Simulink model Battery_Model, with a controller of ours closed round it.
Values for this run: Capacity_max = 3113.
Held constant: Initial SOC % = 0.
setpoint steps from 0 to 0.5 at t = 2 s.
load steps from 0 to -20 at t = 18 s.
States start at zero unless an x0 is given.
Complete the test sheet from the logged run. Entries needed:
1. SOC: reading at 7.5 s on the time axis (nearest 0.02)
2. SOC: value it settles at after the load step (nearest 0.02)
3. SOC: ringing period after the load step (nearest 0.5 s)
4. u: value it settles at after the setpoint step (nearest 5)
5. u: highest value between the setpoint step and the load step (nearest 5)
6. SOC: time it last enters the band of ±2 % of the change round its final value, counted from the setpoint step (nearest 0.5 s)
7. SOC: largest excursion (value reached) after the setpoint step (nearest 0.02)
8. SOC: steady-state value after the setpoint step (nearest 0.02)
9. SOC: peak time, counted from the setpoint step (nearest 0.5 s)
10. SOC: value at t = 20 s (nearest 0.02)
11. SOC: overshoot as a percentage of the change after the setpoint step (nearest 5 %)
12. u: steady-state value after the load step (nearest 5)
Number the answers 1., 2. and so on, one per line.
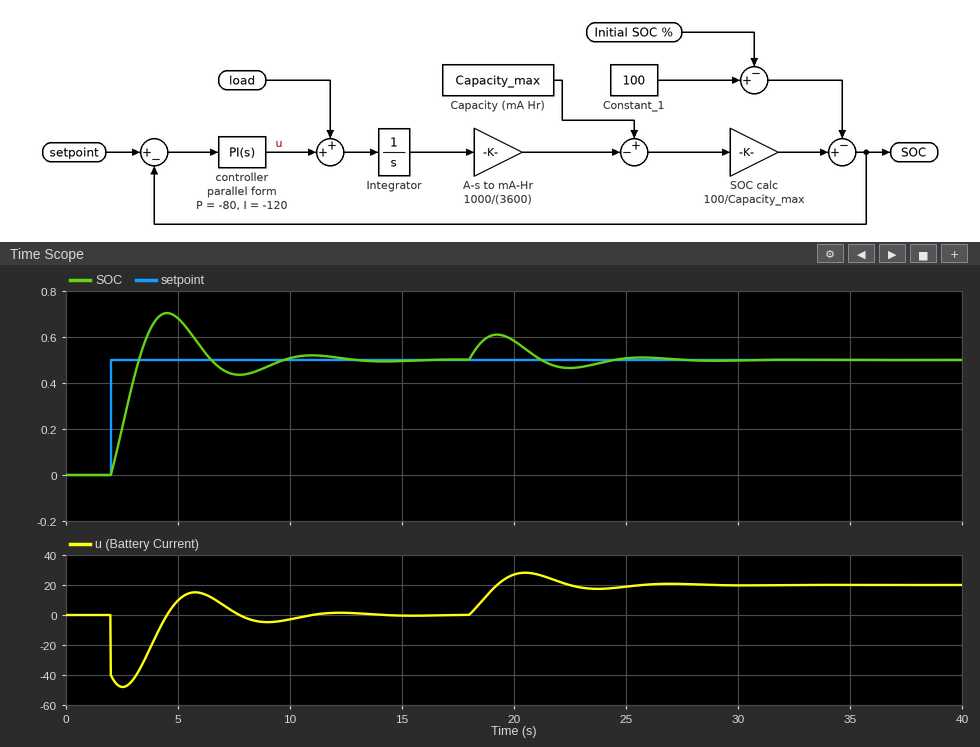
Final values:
1. 0.44
2. 0.50
3. 6.5 s
4. 0
5. 15
6. 10.0 s
7. 0.70
8. 0.50
9. 2.5 s
10. 0.58
11. 40 %
12. 20
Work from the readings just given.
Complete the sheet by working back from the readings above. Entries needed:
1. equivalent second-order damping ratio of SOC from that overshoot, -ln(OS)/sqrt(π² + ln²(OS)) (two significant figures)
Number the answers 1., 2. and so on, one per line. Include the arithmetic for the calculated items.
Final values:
1. ln(0.4) = -0.916; 0.916 / sqrt(9.870 + 0.840) = 0.28
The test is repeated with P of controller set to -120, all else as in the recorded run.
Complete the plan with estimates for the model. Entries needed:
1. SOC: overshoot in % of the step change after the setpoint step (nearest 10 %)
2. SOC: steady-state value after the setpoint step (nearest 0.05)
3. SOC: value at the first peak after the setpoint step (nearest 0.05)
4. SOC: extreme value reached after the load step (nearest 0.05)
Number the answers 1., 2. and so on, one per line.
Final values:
1. 30 %
2. 0.50
3. 0.65
4. 0.60
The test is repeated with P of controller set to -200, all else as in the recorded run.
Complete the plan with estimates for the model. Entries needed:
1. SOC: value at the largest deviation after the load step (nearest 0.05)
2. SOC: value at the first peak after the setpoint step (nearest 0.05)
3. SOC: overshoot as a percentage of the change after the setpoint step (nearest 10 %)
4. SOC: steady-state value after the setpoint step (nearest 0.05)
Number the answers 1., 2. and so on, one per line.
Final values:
1. 0.55
2. 0.60
3. 20 %
4. 0.50
